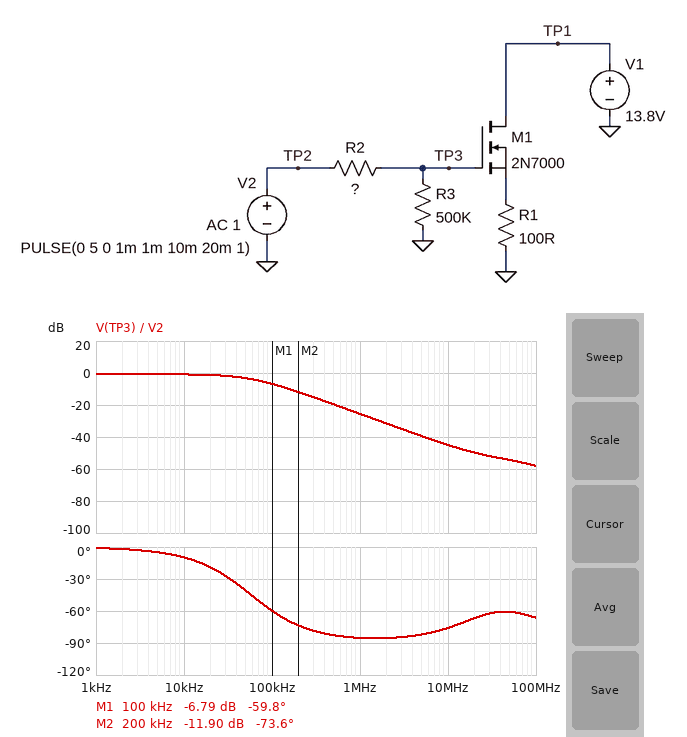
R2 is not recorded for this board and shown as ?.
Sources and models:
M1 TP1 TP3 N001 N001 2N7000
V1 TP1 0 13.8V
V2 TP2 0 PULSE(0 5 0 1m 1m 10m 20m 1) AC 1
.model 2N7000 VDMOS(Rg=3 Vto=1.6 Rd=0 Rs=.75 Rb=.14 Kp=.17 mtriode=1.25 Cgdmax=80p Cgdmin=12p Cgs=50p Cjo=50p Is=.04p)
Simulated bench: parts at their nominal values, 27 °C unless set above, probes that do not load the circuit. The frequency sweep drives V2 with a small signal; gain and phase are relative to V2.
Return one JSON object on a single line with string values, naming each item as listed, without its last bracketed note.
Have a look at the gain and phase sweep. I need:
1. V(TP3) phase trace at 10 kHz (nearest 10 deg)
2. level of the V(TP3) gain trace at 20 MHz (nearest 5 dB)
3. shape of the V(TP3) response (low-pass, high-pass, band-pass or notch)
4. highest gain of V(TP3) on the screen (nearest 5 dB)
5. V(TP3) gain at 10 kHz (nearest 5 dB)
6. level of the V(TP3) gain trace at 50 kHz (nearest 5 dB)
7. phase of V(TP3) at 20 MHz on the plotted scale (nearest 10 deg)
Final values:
{"V(TP3) phase trace at 10 kHz": "-10 deg", "level of the V(TP3) gain trace at 20 MHz": "-50 dB", "shape of the V(TP3) response": "low-pass", "highest gain of V(TP3) on the screen": "0 dB", "V(TP3) gain at 10 kHz": "0 dB", "level of the V(TP3) gain trace at 50 kHz": "-5 dB", "phase of V(TP3) at 20 MHz on the plotted scale": "-70 deg"}
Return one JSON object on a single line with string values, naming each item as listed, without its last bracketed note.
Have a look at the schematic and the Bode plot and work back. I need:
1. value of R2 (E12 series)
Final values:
{"value of R2": "47 kΩ"}
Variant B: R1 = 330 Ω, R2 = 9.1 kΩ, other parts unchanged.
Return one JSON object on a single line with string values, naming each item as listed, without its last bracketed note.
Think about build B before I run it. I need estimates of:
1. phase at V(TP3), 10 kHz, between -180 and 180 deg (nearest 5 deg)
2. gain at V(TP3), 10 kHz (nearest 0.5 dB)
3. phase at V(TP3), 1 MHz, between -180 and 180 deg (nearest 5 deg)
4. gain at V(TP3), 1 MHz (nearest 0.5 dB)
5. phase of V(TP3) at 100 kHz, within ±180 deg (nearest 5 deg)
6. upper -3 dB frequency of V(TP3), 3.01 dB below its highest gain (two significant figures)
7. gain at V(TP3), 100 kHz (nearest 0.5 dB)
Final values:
{"phase at V(TP3), 10 kHz, between -180 and 180 deg": "0 deg", "gain at V(TP3), 10 kHz": "0 dB", "phase at V(TP3), 1 MHz, between -180 and 180 deg": "-70 deg", "gain at V(TP3), 1 MHz": "-11.5 dB", "phase of V(TP3) at 100 kHz, within ±180 deg": "-20 deg", "upper -3 dB frequency of V(TP3), 3.01 dB below its highest gain": "270 kHz", "gain at V(TP3), 100 kHz": "-0.5 dB"}
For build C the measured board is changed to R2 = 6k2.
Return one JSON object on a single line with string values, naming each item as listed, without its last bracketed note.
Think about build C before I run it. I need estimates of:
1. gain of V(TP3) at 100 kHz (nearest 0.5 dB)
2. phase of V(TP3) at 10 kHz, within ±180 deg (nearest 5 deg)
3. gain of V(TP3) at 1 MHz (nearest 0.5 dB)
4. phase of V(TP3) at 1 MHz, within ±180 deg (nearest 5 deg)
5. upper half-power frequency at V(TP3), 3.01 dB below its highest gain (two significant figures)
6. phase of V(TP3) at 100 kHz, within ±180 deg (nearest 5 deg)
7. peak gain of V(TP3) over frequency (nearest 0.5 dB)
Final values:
{"gain of V(TP3) at 100 kHz": "-0.5 dB", "phase of V(TP3) at 10 kHz, within ±180 deg": "0 deg", "gain of V(TP3) at 1 MHz": "-8.5 dB", "phase of V(TP3) at 1 MHz, within ±180 deg": "-65 deg", "upper half-power frequency at V(TP3), 3.01 dB below its highest gain": "400 kHz", "phase of V(TP3) at 100 kHz, within ±180 deg": "-15 deg", "peak gain of V(TP3) over frequency": "0 dB"}
